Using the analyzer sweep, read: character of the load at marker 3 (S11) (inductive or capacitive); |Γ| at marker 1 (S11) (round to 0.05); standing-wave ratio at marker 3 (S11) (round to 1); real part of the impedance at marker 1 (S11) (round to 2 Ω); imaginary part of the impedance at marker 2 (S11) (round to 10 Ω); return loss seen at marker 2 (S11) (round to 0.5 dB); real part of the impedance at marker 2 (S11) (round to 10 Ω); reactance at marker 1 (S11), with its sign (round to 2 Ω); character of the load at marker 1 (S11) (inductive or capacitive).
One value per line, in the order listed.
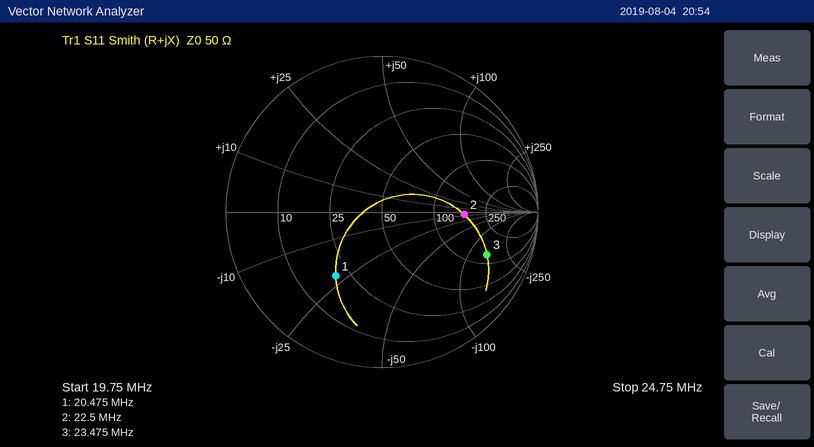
capacitive
0.50
6
20 Ω
-10 Ω
5.5 dB
160 Ω
-22 Ω
capacitive
